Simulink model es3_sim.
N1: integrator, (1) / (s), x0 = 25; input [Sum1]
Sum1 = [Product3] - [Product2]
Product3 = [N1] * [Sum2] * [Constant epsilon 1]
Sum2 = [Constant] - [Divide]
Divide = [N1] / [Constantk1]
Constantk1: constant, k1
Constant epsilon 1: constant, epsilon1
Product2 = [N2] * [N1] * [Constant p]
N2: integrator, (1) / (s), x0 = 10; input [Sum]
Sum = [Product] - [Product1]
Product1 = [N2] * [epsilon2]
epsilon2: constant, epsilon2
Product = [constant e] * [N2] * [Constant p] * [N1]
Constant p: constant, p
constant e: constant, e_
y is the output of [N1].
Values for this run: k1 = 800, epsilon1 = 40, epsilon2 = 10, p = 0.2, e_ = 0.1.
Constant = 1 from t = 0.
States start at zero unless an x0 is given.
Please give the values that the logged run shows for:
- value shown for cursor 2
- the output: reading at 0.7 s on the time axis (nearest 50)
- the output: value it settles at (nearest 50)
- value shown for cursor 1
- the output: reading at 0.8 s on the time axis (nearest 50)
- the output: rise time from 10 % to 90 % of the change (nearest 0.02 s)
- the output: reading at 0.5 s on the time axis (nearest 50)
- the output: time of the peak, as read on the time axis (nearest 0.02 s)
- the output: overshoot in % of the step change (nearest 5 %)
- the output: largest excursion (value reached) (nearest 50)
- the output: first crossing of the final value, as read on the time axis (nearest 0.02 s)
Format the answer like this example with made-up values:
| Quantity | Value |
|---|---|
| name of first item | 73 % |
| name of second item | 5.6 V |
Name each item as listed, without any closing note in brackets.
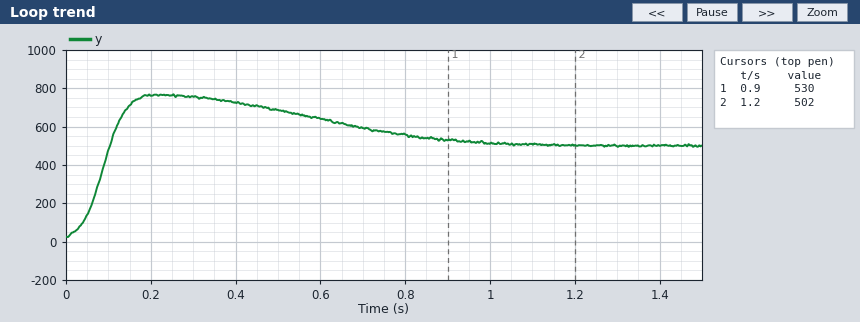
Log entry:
| Quantity | Value |
|---|---|
| value shown for cursor 2 | 502 |
| the output: reading at 0.7 s on the time axis | 600 |
| the output: value it settles at | 500 |
| value shown for cursor 1 | 530 |
| the output: reading at 0.8 s on the time axis | 550 |
| the output: rise time from 10 % to 90 % of the change | 0.06 s |
| the output: reading at 0.5 s on the time axis | 700 |
| the output: time of the peak, as read on the time axis | 0.22 s |
| the output: overshoot in % of the step change | 55 % |
| the output: largest excursion (value reached) | 750 |
| the output: first crossing of the final value, as read on the time axis | 0.10 s |
